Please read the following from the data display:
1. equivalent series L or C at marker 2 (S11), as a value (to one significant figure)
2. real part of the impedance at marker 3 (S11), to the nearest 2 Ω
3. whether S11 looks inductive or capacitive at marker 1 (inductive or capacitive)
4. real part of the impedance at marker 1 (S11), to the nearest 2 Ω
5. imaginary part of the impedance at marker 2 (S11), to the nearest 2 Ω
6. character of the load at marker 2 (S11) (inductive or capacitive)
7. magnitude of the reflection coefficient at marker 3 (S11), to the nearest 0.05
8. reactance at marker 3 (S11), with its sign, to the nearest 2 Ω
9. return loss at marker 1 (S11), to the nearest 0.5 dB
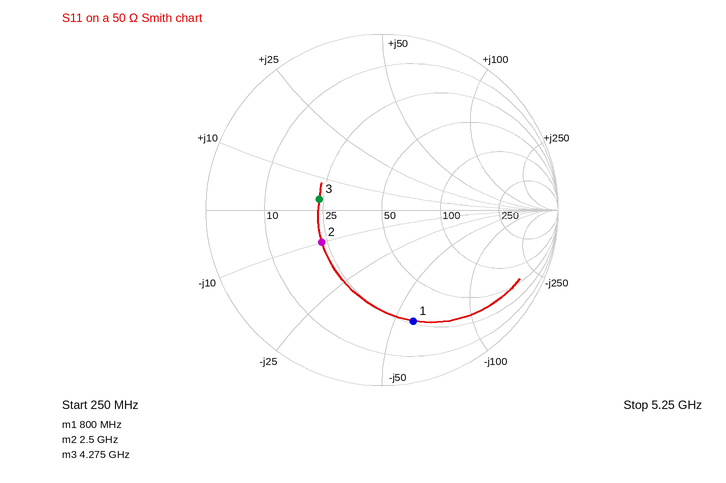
6 pF
24 Ω
capacitive
26 Ω
-10 Ω
capacitive
0.35
+4 Ω
3.5 dB
